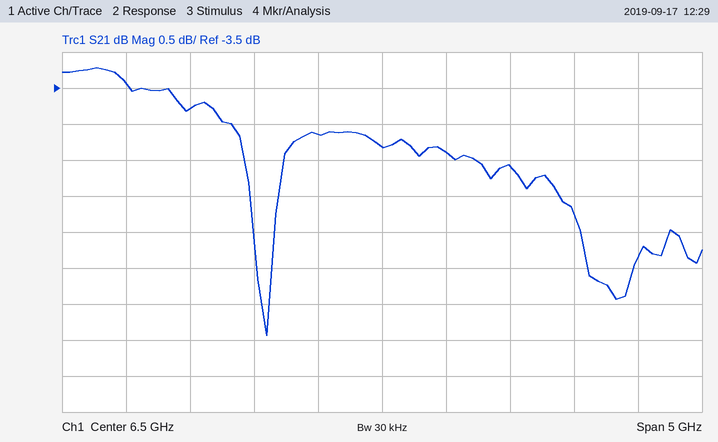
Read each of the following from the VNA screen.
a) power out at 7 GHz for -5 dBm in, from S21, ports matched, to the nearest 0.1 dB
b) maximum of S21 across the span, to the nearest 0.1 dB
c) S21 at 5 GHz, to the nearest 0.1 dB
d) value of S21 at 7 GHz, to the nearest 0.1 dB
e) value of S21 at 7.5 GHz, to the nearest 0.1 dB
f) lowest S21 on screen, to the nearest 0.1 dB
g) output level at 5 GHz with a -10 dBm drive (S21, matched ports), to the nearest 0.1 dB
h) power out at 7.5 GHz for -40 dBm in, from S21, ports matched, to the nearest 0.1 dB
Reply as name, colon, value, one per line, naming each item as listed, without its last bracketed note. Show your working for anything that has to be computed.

power out at 7 GHz for -5 dBm in, from S21, ports matched, to the nearest 0.1 dB: -5 dBm + (-4.4 dB) = -9.4 dBm
maximum of S21 across the span, to the nearest 0.1 dB: -3.2 dB
S21 at 5 GHz, to the nearest 0.1 dB: -3.8 dB
value of S21 at 7 GHz, to the nearest 0.1 dB: -4.4 dB
value of S21 at 7.5 GHz, to the nearest 0.1 dB: -4.6 dB
lowest S21 on screen, to the nearest 0.1 dB: -6.9 dB
output level at 5 GHz with a -10 dBm drive (S21, matched ports), to the nearest 0.1 dB: -10 dBm + (-3.8 dB) = -13.8 dBm
power out at 7.5 GHz for -40 dBm in, from S21, ports matched, to the nearest 0.1 dB: -40 dBm + (-4.6 dB) = -44.6 dBm
